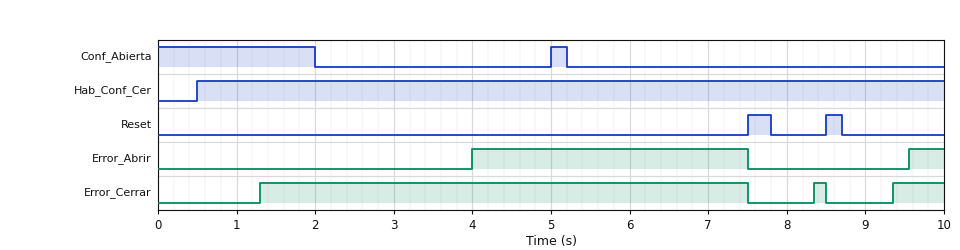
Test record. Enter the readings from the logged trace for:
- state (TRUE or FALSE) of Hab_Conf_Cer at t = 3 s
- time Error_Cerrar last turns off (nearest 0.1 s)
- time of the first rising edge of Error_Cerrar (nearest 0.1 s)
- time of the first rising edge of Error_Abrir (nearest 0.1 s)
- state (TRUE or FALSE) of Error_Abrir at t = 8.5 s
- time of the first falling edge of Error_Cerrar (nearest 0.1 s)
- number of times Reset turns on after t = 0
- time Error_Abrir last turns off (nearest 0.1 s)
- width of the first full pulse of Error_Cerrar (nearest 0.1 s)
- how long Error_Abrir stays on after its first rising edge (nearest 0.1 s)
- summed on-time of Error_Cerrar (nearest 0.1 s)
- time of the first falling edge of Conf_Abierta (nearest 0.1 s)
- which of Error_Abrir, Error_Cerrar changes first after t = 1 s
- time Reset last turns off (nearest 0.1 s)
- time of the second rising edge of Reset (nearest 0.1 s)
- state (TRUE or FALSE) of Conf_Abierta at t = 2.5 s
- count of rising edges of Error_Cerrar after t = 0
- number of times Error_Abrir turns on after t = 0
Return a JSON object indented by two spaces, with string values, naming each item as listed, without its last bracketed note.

{
  "state (TRUE or FALSE) of Hab_Conf_Cer at t = 3 s": "TRUE",
  "time Error_Cerrar last turns off": "8.5 s",
  "time of the first rising edge of Error_Cerrar": "1.3 s",
  "time of the first rising edge of Error_Abrir": "4.0 s",
  "state (TRUE or FALSE) of Error_Abrir at t = 8.5 s": "FALSE",
  "time of the first falling edge of Error_Cerrar": "7.5 s",
  "number of times Reset turns on after t = 0": "2",
  "time Error_Abrir last turns off": "7.5 s",
  "width of the first full pulse of Error_Cerrar": "6.2 s",
  "how long Error_Abrir stays on after its first rising edge": "3.5 s",
  "summed on-time of Error_Cerrar": "7.0 s",
  "time of the first falling edge of Conf_Abierta": "2.0 s",
  "which of Error_Abrir, Error_Cerrar changes first after t = 1 s": "Error_Cerrar",
  "time Reset last turns off": "8.7 s",
  "time of the second rising edge of Reset": "8.5 s",
  "state (TRUE or FALSE) of Conf_Abierta at t = 2.5 s": "FALSE",
  "count of rising edges of Error_Cerrar after t = 0": "3",
  "number of times Error_Abrir turns on after t = 0": "2"
}
